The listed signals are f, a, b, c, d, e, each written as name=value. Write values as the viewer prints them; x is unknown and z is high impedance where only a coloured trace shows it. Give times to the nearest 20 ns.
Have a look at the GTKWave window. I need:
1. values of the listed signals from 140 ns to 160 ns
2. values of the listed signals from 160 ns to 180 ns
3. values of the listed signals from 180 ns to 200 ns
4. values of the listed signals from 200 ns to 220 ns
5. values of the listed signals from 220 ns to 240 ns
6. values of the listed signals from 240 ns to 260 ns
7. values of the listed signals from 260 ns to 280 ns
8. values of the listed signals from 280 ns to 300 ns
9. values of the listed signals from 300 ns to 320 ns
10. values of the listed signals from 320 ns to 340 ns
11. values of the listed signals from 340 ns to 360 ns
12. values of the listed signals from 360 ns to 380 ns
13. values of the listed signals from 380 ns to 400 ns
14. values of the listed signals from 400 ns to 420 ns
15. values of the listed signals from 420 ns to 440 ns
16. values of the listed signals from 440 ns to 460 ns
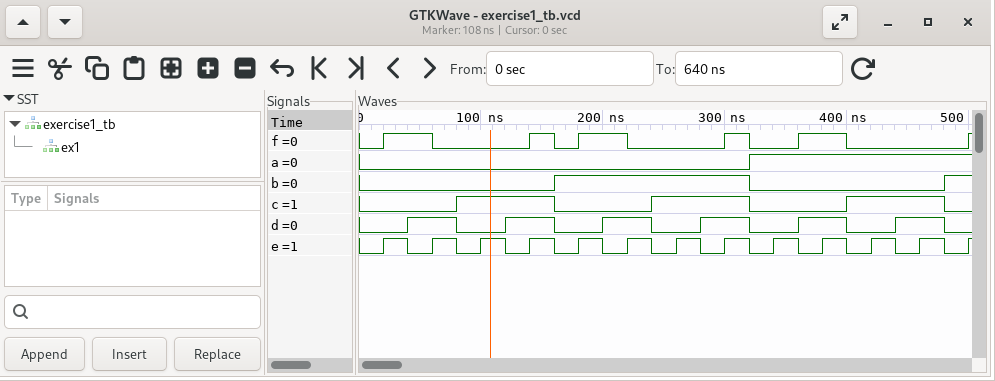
f=1, a=0, b=0, c=1, d=1, e=1
f=0, a=0, b=1, c=0, d=0, e=0
f=1, a=0, b=1, c=0, d=0, e=1
f=1, a=0, b=1, c=0, d=1, e=0
f=0, a=0, b=1, c=0, d=1, e=1
f=0, a=0, b=1, c=1, d=0, e=0
f=0, a=0, b=1, c=1, d=0, e=1
f=0, a=0, b=1, c=1, d=1, e=0
f=1, a=0, b=1, c=1, d=1, e=1
f=0, a=1, b=0, c=0, d=0, e=0
f=0, a=1, b=0, c=0, d=0, e=1
f=1, a=1, b=0, c=0, d=1, e=0
f=1, a=1, b=0, c=0, d=1, e=1
f=0, a=1, b=0, c=1, d=0, e=0
f=0, a=1, b=0, c=1, d=0, e=1
f=0, a=1, b=0, c=1, d=1, e=0
